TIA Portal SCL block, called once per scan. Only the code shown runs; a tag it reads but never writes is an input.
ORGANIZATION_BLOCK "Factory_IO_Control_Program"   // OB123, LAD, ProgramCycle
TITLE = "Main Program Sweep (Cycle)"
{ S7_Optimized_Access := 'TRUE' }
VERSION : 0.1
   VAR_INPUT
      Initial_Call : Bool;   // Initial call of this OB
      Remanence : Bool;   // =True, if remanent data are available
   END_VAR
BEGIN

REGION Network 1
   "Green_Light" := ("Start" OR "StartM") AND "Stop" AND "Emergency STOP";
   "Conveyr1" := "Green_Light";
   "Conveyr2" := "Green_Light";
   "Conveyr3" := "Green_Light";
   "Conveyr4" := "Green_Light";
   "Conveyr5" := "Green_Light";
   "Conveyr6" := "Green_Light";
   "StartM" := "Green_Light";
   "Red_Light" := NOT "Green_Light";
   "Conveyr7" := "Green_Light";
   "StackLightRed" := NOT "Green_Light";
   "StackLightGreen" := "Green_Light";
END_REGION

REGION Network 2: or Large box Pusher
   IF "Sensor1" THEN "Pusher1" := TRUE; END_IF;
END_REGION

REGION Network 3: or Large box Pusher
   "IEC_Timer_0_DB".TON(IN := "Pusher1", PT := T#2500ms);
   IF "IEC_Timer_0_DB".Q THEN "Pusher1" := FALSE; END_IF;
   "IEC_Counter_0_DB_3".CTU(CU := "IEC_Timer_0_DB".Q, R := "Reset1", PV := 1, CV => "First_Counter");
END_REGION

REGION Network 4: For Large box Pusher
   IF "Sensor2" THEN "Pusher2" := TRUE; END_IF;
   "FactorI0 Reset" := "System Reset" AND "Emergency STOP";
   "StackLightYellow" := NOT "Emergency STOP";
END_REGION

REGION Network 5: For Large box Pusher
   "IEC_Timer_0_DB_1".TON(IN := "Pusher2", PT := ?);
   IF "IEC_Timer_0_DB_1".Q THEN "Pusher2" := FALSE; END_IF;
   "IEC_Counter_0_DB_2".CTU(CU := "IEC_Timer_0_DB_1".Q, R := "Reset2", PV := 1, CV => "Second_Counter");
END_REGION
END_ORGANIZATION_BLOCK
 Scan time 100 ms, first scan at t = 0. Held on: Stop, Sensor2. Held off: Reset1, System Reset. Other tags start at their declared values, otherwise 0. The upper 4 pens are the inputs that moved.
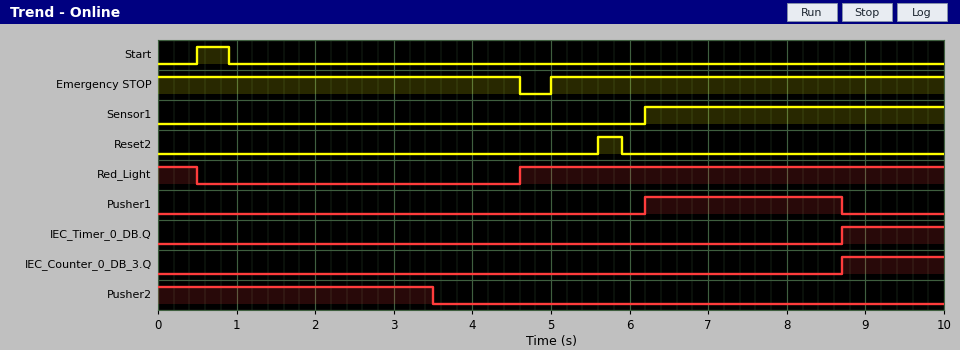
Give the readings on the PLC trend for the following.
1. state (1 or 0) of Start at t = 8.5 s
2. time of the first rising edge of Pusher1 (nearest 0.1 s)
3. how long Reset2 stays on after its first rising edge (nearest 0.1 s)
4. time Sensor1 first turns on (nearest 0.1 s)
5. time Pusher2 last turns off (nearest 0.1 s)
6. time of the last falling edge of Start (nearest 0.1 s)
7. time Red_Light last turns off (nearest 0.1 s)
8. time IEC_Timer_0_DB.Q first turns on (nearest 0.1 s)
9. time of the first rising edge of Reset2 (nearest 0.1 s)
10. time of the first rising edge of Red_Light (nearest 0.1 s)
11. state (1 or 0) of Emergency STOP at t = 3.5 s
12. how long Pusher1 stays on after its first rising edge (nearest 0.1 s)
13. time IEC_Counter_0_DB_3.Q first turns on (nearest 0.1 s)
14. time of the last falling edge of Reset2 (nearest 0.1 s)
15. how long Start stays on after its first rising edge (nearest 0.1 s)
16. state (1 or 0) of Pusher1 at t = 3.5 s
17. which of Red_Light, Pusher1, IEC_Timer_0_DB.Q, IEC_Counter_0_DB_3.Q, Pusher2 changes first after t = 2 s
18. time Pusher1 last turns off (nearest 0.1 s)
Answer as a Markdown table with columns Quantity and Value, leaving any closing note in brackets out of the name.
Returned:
| Quantity | Value |
|---|---|
| state (1 or 0) of Start at t = 8.5 s | 0 |
| time of the first rising edge of Pusher1 | 6.2 s |
| how long Reset2 stays on after its first rising edge | 0.3 s |
| time Sensor1 first turns on | 6.2 s |
| time Pusher2 last turns off | 3.5 s |
| time of the last falling edge of Start | 0.9 s |
| time Red_Light last turns off | 0.5 s |
| time IEC_Timer_0_DB.Q first turns on | 8.7 s |
| time of the first rising edge of Reset2 | 5.6 s |
| time of the first rising edge of Red_Light | 4.6 s |
| state (1 or 0) of Emergency STOP at t = 3.5 s | 1 |
| how long Pusher1 stays on after its first rising edge | 2.5 s |
| time IEC_Counter_0_DB_3.Q first turns on | 8.7 s |
| time of the last falling edge of Reset2 | 5.9 s |
| how long Start stays on after its first rising edge | 0.4 s |
| state (1 or 0) of Pusher1 at t = 3.5 s | 0 |
| which of Red_Light, Pusher1, IEC_Timer_0_DB.Q, IEC_Counter_0_DB_3.Q, Pusher2 changes first after t = 2 s | Pusher2 |
| time Pusher1 last turns off | 8.7 s |
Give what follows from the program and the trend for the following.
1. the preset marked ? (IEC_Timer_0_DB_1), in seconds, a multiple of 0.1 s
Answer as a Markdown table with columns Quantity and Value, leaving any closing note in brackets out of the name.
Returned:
| Quantity | Value |
|---|---|
| the preset marked ? (IEC_Timer_0_DB_1), in seconds, a multiple of 0.1 s | 3.5 s |
